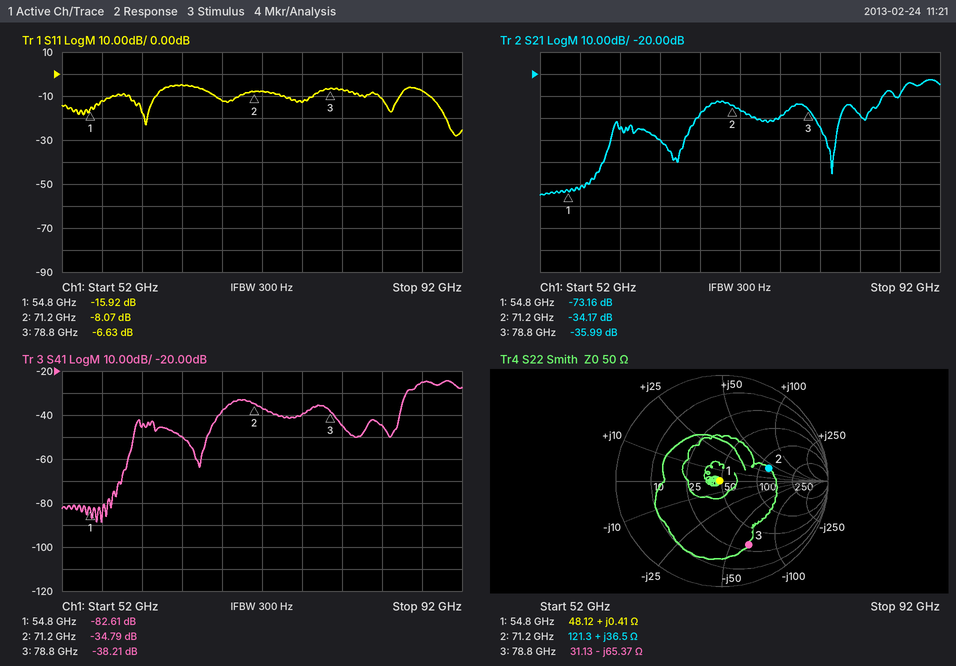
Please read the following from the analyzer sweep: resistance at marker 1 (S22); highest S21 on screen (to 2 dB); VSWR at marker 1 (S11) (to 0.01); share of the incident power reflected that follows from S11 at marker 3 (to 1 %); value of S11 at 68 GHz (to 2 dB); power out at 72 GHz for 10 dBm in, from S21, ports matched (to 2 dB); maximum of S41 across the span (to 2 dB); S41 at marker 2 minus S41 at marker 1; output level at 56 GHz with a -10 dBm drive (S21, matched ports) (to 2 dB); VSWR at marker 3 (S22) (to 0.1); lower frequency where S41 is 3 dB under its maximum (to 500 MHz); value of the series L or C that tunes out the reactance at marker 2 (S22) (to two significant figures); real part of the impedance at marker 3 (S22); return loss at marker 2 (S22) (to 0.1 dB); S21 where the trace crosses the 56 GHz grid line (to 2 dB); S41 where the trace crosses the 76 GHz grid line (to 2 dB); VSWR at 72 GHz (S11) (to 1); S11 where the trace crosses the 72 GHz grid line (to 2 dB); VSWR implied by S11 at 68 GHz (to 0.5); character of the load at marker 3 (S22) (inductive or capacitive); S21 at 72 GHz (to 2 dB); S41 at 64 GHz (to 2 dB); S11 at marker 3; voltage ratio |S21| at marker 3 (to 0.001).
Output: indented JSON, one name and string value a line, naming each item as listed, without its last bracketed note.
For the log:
{
  "resistance at marker 1": "48.12 Ω",
  "highest S21 on screen": "-22 dB",
  "VSWR at marker 1 (S11)": "1.38",
  "share of the incident power reflected that follows from S11 at marker 3": "22 %",
  "value of S11 at 68 GHz": "-12 dB",
  "power out at 72 GHz for 10 dBm in, from S21, ports matched": "-26 dBm",
  "maximum of S41 across the span": "-24 dB",
  "S41 at marker 2 minus S41 at marker 1": "47.82 dB",
  "output level at 56 GHz with a -10 dBm drive (S21, matched ports)": "-82 dBm",
  "VSWR at marker 3 (S22)": "4.8",
  "lower frequency where S41 is 3 dB under its maximum": "87.5 GHz",
  "value of the series L or C that tunes out the reactance at marker 2 (S22)": "61 fF",
  "real part of the impedance at marker 3": "31.13 Ω",
  "return loss at marker 2 (S22)": "6.8 dB",
  "S21 where the trace crosses the 56 GHz grid line": "-72 dB",
  "S41 where the trace crosses the 76 GHz grid line": "-40 dB",
  "VSWR at 72 GHz (S11)": "2",
  "S11 where the trace crosses the 72 GHz grid line": "-8 dB",
  "VSWR implied by S11 at 68 GHz": "1.5",
  "character of the load at marker 3 (S22)": "capacitive",
  "S21 at 72 GHz": "-36 dB",
  "S41 at 64 GHz": "-50 dB",
  "S11 at marker 3": "-6.63 dB",
  "voltage ratio |S21| at marker 3": "0.016"
}
